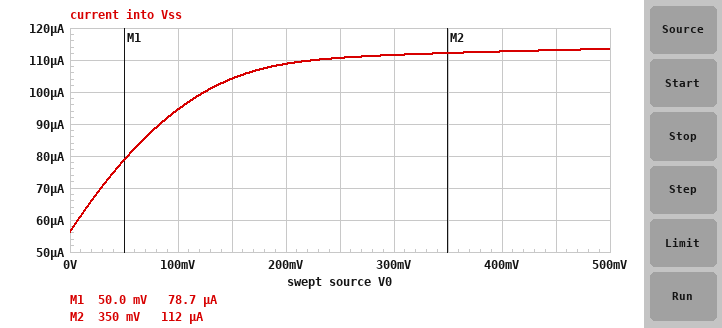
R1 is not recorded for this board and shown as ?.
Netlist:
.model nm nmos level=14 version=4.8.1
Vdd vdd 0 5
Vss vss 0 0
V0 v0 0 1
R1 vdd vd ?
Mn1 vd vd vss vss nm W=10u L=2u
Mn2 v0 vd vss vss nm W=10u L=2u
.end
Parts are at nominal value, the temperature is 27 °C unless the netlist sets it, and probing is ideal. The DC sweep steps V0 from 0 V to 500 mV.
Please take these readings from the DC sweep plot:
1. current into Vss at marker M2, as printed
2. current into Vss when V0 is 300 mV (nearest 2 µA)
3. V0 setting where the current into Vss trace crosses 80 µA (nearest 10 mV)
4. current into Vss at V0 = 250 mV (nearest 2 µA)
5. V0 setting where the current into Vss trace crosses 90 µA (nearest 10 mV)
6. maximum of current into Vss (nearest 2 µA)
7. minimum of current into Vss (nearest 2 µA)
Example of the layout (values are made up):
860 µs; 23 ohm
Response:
112 µA; 112 µA; 50 mV; 110 µA; 80 mV; 114 µA; 56 µA
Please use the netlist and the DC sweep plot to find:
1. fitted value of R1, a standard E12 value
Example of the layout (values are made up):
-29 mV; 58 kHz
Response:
82 kΩ
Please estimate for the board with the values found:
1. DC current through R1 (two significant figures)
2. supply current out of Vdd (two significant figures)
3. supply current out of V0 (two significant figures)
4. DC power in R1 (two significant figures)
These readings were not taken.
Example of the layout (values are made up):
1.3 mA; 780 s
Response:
56 µA; 56 µA; 60 µA; 260 µW
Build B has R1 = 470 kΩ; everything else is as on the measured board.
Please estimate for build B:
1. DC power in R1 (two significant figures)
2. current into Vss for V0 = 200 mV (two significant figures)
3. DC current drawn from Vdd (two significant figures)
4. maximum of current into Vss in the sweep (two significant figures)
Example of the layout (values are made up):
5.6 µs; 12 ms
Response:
48 µW; 20 µA; 10 µA; 21 µA
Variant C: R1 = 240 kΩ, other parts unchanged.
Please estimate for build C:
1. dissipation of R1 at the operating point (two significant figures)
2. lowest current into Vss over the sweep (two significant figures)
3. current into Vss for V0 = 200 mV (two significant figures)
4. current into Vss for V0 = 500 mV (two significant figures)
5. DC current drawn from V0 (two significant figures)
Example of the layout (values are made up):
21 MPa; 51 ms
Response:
92 µW; 20 µA; 39 µA; 40 µA; 22 µA
